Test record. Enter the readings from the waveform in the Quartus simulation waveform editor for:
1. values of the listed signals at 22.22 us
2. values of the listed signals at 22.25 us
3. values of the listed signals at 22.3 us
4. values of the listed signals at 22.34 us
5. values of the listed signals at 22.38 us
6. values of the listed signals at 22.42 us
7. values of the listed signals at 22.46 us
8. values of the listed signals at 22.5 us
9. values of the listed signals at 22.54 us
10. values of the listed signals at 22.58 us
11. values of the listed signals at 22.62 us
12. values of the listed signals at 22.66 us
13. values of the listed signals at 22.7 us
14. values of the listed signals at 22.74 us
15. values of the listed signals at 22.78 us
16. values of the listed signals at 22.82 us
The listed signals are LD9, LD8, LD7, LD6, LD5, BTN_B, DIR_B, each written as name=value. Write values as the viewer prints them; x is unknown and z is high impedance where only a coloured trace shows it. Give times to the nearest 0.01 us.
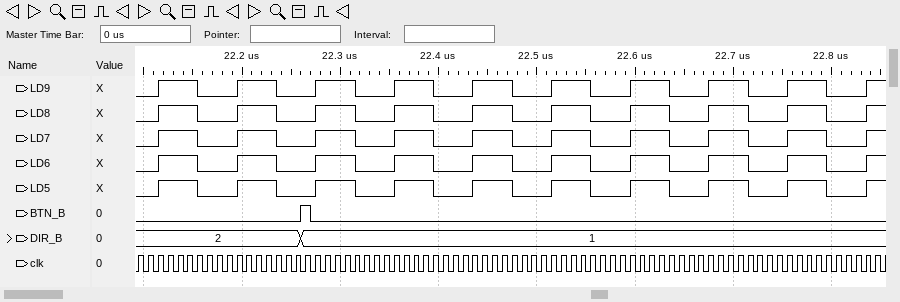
LD9=1, LD8=1, LD7=1, LD6=1, LD5=1, BTN_B=0, DIR_B=2
LD9=0, LD8=0, LD7=0, LD6=0, LD5=0, BTN_B=0, DIR_B=2
LD9=1, LD8=1, LD7=1, LD6=1, LD5=1, BTN_B=0, DIR_B=1
LD9=0, LD8=0, LD7=0, LD6=0, LD5=0, BTN_B=0, DIR_B=1
LD9=1, LD8=1, LD7=1, LD6=1, LD5=1, BTN_B=0, DIR_B=1
LD9=0, LD8=0, LD7=0, LD6=0, LD5=0, BTN_B=0, DIR_B=1
LD9=1, LD8=1, LD7=1, LD6=1, LD5=1, BTN_B=0, DIR_B=1
LD9=0, LD8=0, LD7=0, LD6=0, LD5=0, BTN_B=0, DIR_B=1
LD9=1, LD8=1, LD7=1, LD6=1, LD5=1, BTN_B=0, DIR_B=1
LD9=0, LD8=0, LD7=0, LD6=0, LD5=0, BTN_B=0, DIR_B=1
LD9=1, LD8=1, LD7=1, LD6=1, LD5=1, BTN_B=0, DIR_B=1
LD9=0, LD8=0, LD7=0, LD6=0, LD5=0, BTN_B=0, DIR_B=1
LD9=1, LD8=1, LD7=1, LD6=1, LD5=1, BTN_B=0, DIR_B=1
LD9=0, LD8=0, LD7=0, LD6=0, LD5=0, BTN_B=0, DIR_B=1
LD9=1, LD8=1, LD7=1, LD6=1, LD5=1, BTN_B=0, DIR_B=1
LD9=0, LD8=0, LD7=0, LD6=0, LD5=0, BTN_B=0, DIR_B=1
